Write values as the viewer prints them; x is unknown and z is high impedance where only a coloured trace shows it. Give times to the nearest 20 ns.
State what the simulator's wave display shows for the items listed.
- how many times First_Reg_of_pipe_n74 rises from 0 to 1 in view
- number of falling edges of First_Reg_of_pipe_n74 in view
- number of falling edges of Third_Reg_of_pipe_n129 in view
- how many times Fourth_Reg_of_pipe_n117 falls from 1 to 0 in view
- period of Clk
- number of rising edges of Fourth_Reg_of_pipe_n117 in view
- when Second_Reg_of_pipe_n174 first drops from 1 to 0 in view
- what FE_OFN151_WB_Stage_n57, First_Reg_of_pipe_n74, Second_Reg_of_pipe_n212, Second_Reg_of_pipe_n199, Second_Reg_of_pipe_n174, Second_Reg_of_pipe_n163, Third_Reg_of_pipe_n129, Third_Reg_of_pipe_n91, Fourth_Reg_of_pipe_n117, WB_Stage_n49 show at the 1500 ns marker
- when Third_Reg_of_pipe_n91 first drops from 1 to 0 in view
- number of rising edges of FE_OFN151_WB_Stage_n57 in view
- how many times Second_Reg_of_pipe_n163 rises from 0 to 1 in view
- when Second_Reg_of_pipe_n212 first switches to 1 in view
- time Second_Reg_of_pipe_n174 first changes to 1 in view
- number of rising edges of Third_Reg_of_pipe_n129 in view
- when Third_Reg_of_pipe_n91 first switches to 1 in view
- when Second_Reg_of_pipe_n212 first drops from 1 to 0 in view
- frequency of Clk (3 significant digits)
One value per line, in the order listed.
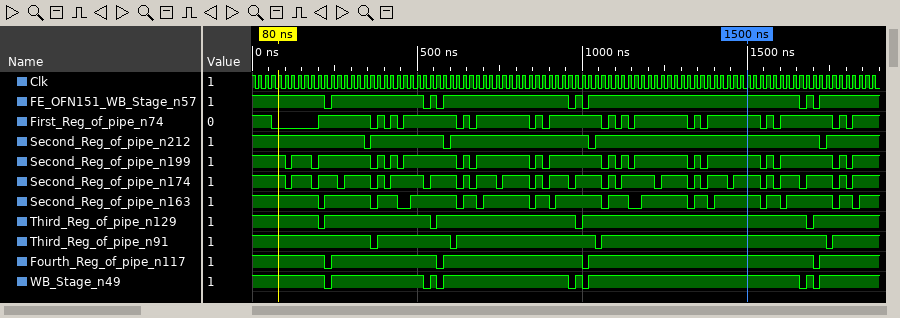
17
17
4
4
20 ns
4
100 ns
FE_OFN151_WB_Stage_n57=1, First_Reg_of_pipe_n74=1, Second_Reg_of_pipe_n212=1, Second_Reg_of_pipe_n199=1, Second_Reg_of_pipe_n174=1, Second_Reg_of_pipe_n163=1, Third_Reg_of_pipe_n129=1, Third_Reg_of_pipe_n91=1, Fourth_Reg_of_pipe_n117=1, WB_Stage_n49=1
360 ns
7
15
360 ns
120 ns
4
380 ns
340 ns
50.0 MHz
